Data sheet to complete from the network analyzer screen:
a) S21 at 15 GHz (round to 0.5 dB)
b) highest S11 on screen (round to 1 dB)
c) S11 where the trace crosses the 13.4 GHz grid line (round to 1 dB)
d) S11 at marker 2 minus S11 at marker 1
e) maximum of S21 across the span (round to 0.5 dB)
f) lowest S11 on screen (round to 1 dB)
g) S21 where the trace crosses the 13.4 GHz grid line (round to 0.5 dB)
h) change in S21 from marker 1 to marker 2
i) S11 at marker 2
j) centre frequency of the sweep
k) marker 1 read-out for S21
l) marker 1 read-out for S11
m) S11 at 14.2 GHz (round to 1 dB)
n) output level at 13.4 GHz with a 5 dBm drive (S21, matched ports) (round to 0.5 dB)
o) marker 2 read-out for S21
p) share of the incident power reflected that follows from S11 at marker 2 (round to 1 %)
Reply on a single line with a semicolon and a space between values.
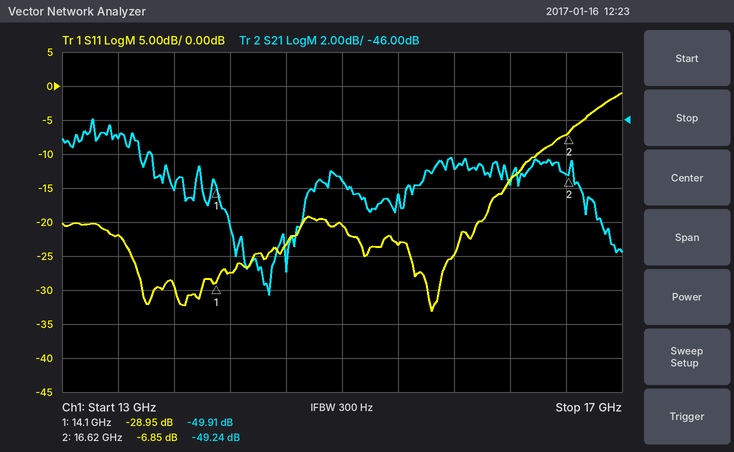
-49.5 dB; -1 dB; -22 dB; 22.10 dB; -46.0 dB; -33 dB; -47.0 dB; 0.67 dB; -6.85 dB; 15 GHz; -49.91 dB; -28.95 dB; -27 dB; -42.0 dBm; -49.24 dB; 21 %
